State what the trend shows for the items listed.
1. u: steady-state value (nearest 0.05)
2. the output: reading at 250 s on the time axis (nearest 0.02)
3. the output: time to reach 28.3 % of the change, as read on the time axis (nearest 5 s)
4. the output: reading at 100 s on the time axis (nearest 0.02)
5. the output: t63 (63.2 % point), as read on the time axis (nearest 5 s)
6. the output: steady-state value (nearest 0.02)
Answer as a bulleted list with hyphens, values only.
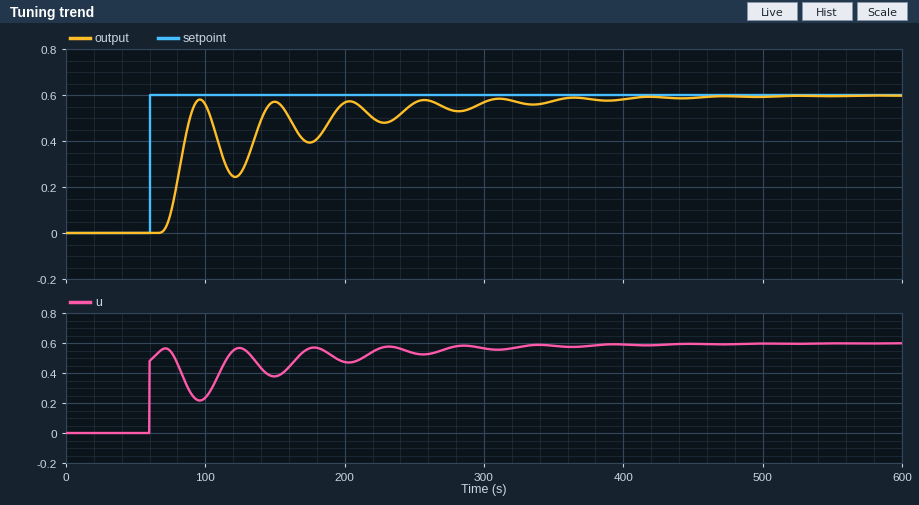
- 0.60
- 0.56
- 80 s
- 0.56
- 85 s
- 0.60
